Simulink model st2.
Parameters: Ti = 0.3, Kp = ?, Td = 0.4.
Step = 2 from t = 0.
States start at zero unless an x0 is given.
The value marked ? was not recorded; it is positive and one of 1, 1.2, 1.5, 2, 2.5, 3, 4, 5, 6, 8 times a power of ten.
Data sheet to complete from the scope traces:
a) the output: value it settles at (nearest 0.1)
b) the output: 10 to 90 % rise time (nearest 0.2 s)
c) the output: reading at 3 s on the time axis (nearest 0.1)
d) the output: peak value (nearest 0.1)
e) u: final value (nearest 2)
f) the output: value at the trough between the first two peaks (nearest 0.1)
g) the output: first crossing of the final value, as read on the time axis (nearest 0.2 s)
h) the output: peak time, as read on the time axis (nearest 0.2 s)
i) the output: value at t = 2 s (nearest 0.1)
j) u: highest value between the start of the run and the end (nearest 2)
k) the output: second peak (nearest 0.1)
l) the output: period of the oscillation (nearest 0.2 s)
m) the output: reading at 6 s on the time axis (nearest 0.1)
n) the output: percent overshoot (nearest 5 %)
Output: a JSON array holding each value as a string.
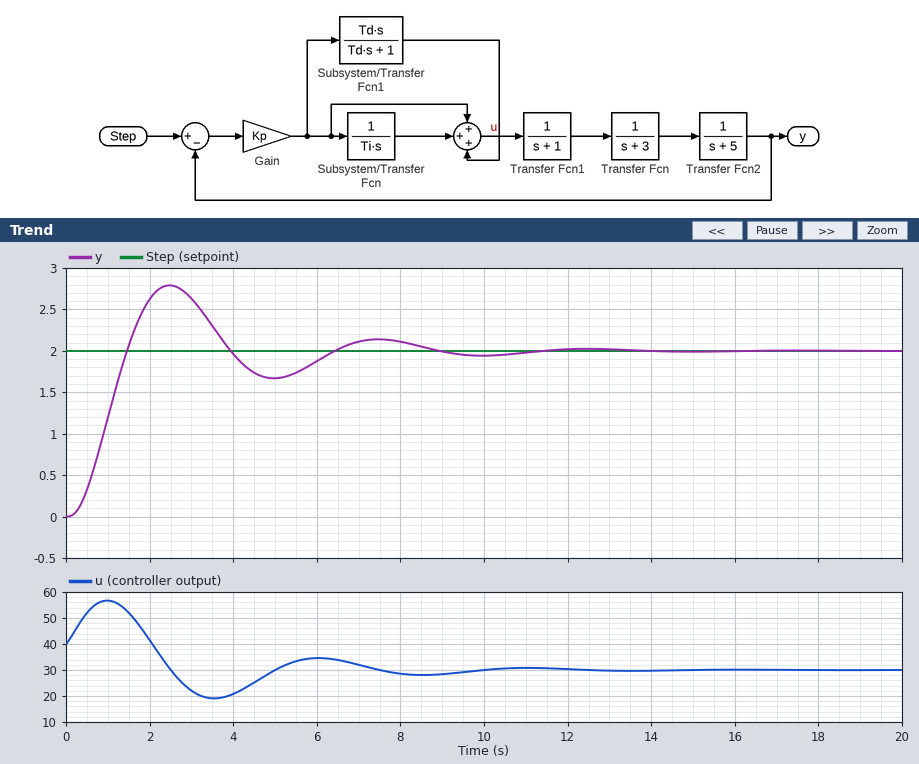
["2.0", "1.0 s", "2.6", "2.8", "30", "1.7", "1.4 s", "2.4 s", "2.6", "56", "2.1", "5.0 s", "1.9", "40 %"]
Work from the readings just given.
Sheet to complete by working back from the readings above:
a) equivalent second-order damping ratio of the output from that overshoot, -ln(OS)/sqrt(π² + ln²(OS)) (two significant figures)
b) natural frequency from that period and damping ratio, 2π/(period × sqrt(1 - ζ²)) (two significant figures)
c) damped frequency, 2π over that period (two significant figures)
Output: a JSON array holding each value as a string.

["0.28", "1.3 rad/s", "1.3 rad/s"]
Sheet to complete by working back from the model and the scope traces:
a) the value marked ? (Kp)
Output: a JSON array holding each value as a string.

["10"]
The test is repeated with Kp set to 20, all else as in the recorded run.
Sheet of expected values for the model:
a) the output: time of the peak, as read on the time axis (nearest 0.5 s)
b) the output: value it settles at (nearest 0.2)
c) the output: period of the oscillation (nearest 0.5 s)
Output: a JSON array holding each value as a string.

["1.5 s", "2.0", "3.5 s"]
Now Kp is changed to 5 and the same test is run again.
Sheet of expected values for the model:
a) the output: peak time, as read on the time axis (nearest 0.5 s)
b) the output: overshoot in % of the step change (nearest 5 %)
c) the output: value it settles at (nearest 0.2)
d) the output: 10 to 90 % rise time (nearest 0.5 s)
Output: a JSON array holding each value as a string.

["3.5 s", "25 %", "2.0", "1.5 s"]
